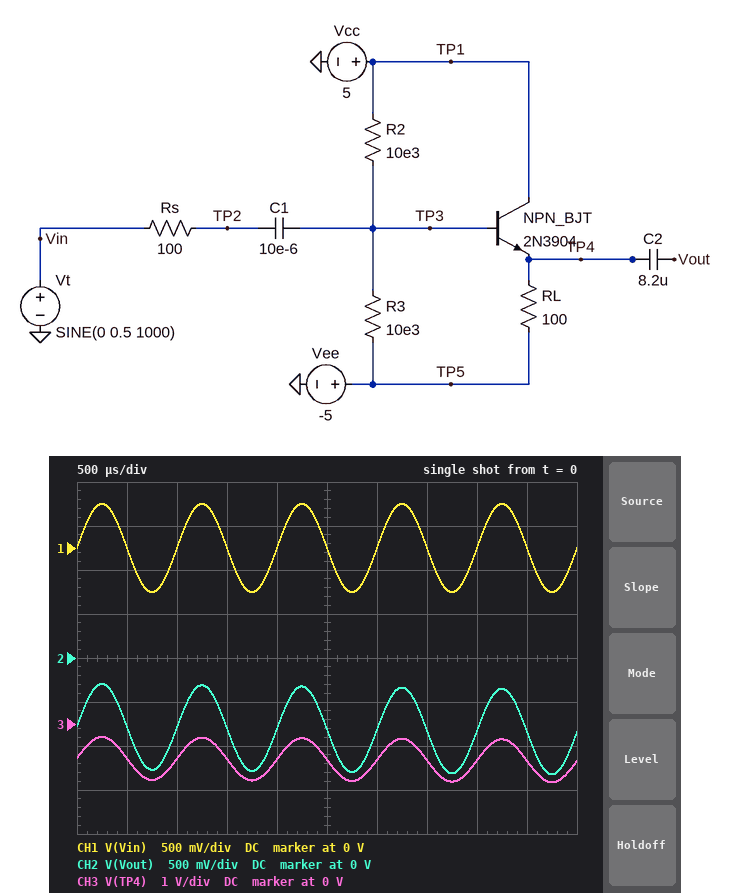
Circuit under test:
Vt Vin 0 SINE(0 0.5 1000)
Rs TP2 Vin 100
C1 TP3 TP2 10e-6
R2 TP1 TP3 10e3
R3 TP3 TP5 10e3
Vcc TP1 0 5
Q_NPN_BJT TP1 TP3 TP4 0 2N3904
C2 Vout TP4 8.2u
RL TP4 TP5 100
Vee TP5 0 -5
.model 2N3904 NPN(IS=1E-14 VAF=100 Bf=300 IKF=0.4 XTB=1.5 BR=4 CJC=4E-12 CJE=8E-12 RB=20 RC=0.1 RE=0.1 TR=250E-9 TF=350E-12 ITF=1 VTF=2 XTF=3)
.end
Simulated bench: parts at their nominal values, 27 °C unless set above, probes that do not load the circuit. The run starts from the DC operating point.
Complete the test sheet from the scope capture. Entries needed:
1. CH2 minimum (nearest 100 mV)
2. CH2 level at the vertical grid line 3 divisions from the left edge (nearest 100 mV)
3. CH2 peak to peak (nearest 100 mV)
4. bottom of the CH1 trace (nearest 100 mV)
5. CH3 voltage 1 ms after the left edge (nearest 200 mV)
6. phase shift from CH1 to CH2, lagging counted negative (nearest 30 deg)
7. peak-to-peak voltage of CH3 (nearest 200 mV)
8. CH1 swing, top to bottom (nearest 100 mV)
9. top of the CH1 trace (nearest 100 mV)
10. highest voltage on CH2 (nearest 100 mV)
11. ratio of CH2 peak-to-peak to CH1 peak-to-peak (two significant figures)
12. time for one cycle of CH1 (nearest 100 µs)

-1.3 V
-800 mV
1.0 V
-500 mV
-800 mV
0 deg
1.0 V
1.0 V
500 mV
-300 mV
1.0
1.0 ms
